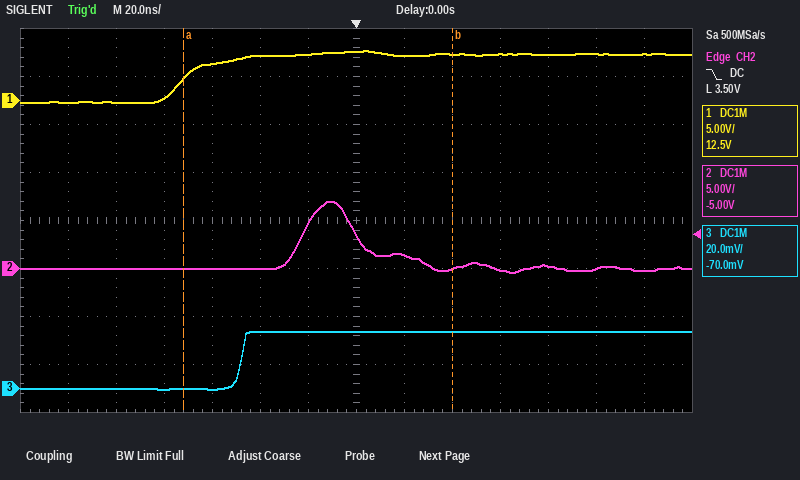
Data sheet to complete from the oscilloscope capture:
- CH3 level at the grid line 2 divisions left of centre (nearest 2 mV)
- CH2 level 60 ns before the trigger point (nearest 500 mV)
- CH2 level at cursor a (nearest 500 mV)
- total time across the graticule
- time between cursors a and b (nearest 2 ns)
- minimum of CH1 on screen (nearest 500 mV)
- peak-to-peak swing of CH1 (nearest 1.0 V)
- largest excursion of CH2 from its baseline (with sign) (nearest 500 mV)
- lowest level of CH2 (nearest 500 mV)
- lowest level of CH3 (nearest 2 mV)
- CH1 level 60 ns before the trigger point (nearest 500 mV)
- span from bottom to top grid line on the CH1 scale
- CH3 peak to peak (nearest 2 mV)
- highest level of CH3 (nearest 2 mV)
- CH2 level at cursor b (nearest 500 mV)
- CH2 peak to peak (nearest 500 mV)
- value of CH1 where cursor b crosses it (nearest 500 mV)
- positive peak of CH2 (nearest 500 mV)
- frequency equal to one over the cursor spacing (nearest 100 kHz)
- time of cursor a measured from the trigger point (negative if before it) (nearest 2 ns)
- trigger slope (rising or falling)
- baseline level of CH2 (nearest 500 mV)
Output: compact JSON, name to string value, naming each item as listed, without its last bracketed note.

{"CH3 level at the grid line 2 divisions left of centre": "24 mV", "CH2 level 60 ns before the trigger point": "0.0 V", "CH2 level at cursor a": "0.0 V", "total time across the graticule": "280 ns", "time between cursors a and b": "112 ns", "minimum of CH1 on screen": "0.0 V", "peak-to-peak swing of CH1": "5.0 V", "largest excursion of CH2 from its baseline (with sign)": "+7.0 V", "lowest level of CH2": "-500 mV", "lowest level of CH3": "0 mV", "CH1 level 60 ns before the trigger point": "4.0 V", "span from bottom to top grid line on the CH1 scale": "40 V", "CH3 peak to peak": "24 mV", "highest level of CH3": "24 mV", "CH2 level at cursor b": "0.0 V", "CH2 peak to peak": "7.5 V", "value of CH1 where cursor b crosses it": "5.0 V", "positive peak of CH2": "7.0 V", "frequency equal to one over the cursor spacing": "8.9 MHz", "time of cursor a measured from the trigger point (negative if before it)": "-72 ns", "trigger slope": "falling", "baseline level of CH2": "0.0 V"}
